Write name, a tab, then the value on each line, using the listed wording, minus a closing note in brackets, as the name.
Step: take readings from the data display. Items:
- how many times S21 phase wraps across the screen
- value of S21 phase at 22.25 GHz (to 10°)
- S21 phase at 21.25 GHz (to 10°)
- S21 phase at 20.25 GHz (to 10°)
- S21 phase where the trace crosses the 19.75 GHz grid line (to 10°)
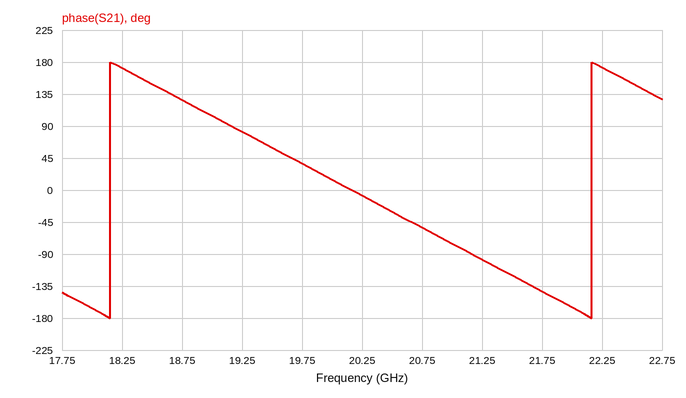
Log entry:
how many times S21 phase wraps across the screen	2
value of S21 phase at 22.25 GHz	170°
S21 phase at 21.25 GHz	-100°
S21 phase at 20.25 GHz	-10°
S21 phase where the trace crosses the 19.75 GHz grid line	40°
